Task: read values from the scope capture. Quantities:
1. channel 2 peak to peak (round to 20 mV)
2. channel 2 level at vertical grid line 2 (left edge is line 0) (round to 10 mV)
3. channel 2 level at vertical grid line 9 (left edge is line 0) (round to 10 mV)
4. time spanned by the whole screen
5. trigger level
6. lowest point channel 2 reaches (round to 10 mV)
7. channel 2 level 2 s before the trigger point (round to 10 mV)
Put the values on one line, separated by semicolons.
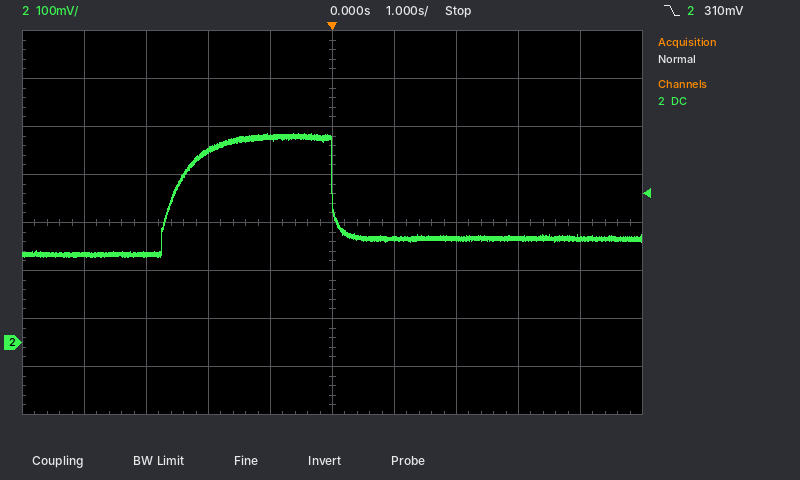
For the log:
260 mV; 180 mV; 220 mV; 10 s; 310 mV; 180 mV; 400 mV
